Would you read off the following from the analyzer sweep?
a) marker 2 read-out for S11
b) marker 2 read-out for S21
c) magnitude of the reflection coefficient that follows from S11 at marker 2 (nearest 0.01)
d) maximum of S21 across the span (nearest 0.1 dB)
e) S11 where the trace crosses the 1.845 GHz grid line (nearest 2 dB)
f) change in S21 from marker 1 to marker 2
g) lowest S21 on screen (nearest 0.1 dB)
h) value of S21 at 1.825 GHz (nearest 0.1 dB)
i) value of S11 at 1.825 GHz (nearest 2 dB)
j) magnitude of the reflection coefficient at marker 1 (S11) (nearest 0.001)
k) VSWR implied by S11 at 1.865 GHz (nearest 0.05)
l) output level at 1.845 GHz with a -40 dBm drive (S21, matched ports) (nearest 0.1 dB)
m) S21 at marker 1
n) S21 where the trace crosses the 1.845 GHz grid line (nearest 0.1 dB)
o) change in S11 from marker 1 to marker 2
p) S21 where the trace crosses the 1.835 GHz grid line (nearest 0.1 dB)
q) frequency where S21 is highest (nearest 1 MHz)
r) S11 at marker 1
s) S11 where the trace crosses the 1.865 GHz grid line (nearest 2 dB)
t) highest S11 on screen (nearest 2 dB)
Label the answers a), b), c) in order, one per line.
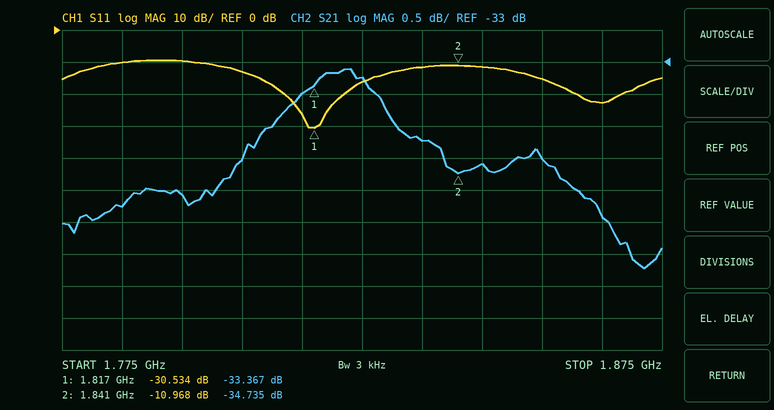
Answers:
a) -10.968 dB
b) -34.735 dB
c) 0.28
d) -33.1 dB
e) -12 dB
f) -1.368 dB
g) -36.2 dB
h) -33.2 dB
i) -16 dB
j) 0.030
k) 1.15
l) -74.6 dBm
m) -33.367 dB
n) -34.6 dB
o) 19.566 dB
p) -34.2 dB
q) 1.823 GHz
r) -30.534 dB
s) -22 dB
t) -10 dB
